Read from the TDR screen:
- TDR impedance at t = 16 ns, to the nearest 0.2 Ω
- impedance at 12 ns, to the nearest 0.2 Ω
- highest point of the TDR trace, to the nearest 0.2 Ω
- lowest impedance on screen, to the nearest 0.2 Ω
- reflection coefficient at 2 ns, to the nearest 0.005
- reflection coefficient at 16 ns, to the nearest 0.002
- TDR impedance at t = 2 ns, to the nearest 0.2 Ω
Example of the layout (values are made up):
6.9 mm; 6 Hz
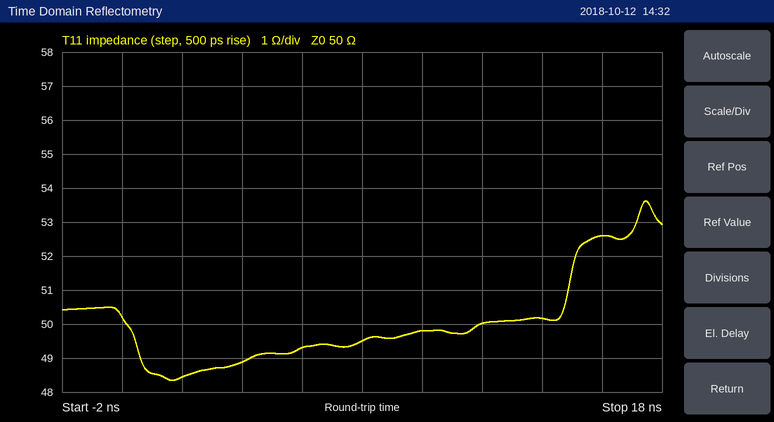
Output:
52.6 Ω; 50.0 Ω; 53.6 Ω; 48.4 Ω; -0.015; +0.026; 48.4 Ω
